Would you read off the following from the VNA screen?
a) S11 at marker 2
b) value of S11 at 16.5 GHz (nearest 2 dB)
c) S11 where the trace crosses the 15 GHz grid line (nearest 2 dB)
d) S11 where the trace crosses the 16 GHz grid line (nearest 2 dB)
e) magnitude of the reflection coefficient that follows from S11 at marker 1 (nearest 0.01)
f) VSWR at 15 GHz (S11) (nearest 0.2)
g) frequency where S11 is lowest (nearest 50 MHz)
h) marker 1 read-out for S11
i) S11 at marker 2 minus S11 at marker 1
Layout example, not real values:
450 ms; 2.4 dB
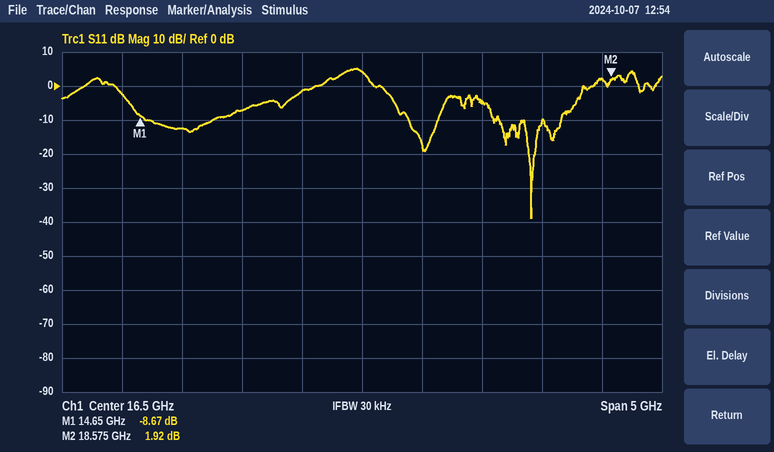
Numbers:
1.92 dB; 4 dB; -12 dB; -2 dB; 0.37; 1.6; 17.90 GHz; -8.67 dB; 10.59 dB
